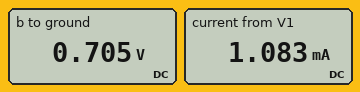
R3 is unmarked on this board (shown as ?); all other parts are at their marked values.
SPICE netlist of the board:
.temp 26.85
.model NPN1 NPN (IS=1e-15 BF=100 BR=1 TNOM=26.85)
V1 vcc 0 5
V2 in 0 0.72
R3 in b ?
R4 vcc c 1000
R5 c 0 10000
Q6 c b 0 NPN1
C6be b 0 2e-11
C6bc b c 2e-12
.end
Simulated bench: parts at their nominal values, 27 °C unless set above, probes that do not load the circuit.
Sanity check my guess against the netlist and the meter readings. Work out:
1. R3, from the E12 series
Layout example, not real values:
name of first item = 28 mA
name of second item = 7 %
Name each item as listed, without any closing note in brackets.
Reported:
R3, from the E12 series = 2.2 kΩ
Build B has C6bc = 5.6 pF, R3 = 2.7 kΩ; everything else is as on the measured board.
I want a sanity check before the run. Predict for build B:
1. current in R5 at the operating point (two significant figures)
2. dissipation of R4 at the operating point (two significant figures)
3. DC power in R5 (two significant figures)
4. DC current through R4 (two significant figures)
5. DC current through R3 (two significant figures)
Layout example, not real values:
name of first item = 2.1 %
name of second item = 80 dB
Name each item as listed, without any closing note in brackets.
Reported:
current in R5 at the operating point = 400 µA
dissipation of R4 at the operating point = 1.1 mW
DC power in R5 = 1.6 mW
DC current through R4 = 1.0 mA
DC current through R3 = 6.4 µA
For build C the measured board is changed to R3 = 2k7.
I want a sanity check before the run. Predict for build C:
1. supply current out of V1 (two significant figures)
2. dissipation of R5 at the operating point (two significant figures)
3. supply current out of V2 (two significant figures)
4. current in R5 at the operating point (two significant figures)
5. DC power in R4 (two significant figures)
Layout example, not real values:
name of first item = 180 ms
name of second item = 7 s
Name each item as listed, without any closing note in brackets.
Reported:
supply current out of V1 = 1.0 mA
dissipation of R5 at the operating point = 1.6 mW
supply current out of V2 = 6.4 µA
current in R5 at the operating point = 400 µA
DC power in R4 = 1.1 mW
